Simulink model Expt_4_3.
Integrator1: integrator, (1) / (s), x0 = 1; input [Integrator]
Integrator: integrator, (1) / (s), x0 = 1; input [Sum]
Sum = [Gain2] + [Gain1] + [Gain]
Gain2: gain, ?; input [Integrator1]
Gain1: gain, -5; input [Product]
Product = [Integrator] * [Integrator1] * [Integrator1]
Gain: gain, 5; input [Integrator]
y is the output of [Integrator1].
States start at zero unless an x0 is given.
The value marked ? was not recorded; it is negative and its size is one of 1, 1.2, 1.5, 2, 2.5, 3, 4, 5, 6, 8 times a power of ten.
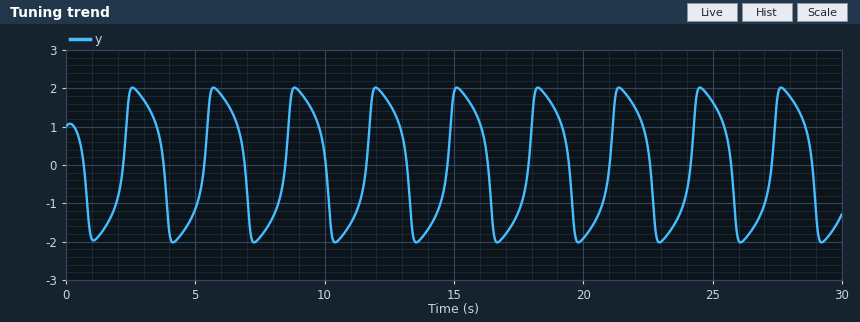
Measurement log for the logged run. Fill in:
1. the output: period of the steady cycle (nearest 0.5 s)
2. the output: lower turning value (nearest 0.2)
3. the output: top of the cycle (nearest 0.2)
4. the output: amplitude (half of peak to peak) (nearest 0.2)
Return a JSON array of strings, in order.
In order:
["3.0 s", "-2.0", "2.0", "2.0"]
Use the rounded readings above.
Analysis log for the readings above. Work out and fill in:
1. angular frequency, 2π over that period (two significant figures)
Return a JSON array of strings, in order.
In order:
["2.1 rad/s"]
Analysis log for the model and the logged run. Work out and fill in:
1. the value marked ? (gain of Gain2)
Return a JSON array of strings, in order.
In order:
["-6"]
